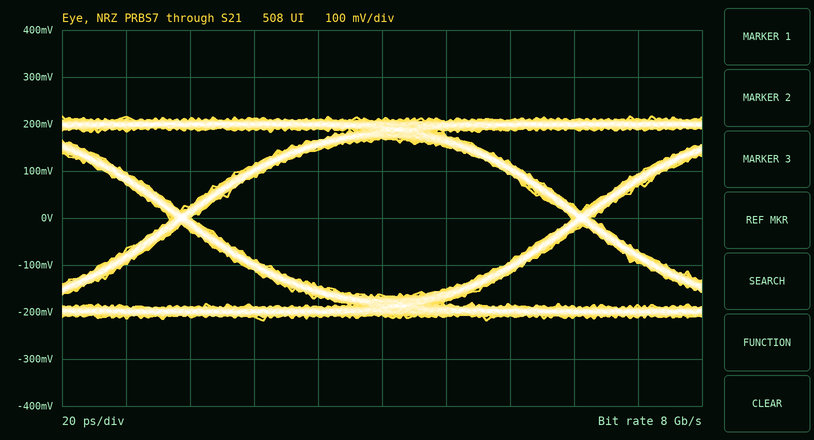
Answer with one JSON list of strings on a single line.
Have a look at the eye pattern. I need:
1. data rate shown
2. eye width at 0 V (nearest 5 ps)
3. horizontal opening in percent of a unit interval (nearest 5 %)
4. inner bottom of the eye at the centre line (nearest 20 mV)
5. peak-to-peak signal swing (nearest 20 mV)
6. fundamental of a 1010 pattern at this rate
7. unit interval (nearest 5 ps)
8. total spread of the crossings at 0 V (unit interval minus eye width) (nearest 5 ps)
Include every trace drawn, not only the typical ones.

["8 Gb/s", "120 ps", "95 %", "-160 mV", "440 mV", "4 GHz", "125 ps", "5 ps"]
